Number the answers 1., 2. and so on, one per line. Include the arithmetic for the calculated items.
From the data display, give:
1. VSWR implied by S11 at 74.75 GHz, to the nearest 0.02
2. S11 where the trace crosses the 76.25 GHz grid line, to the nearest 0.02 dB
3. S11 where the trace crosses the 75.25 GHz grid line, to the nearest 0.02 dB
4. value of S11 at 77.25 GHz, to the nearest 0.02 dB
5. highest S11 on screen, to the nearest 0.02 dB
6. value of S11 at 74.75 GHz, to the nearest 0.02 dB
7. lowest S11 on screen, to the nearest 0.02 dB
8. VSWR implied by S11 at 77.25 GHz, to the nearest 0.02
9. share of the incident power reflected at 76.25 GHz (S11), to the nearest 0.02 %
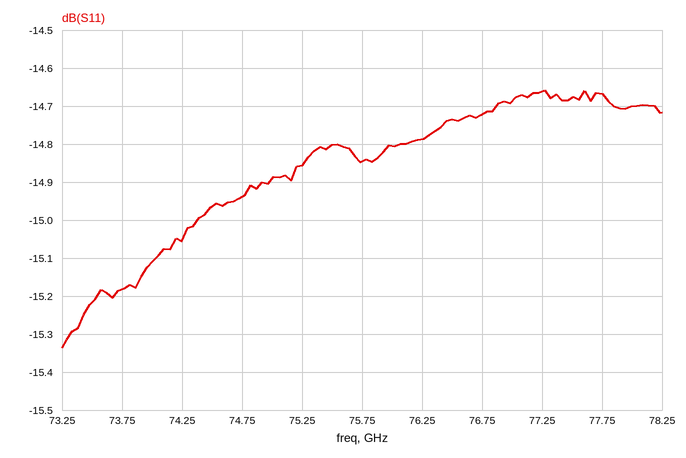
1. |Γ| = 10^(-14.94/20) = 0.1791; VSWR = (1 + 0.1791)/(1 − 0.1791) ≈ 1.44
2. -14.78 dB
3. -14.86 dB
4. -14.66 dB
5. -14.66 dB
6. -14.94 dB
7. -15.34 dB
8. |Γ| = 10^(-14.66/20) = 0.1849; VSWR = (1 + 0.1849)/(1 − 0.1849) ≈ 1.45, so 1.46 to the nearest 0.02
9. 10^(-14.78/10) ≈ 3.33 %, so 3.32 % to the nearest 0.02 %
